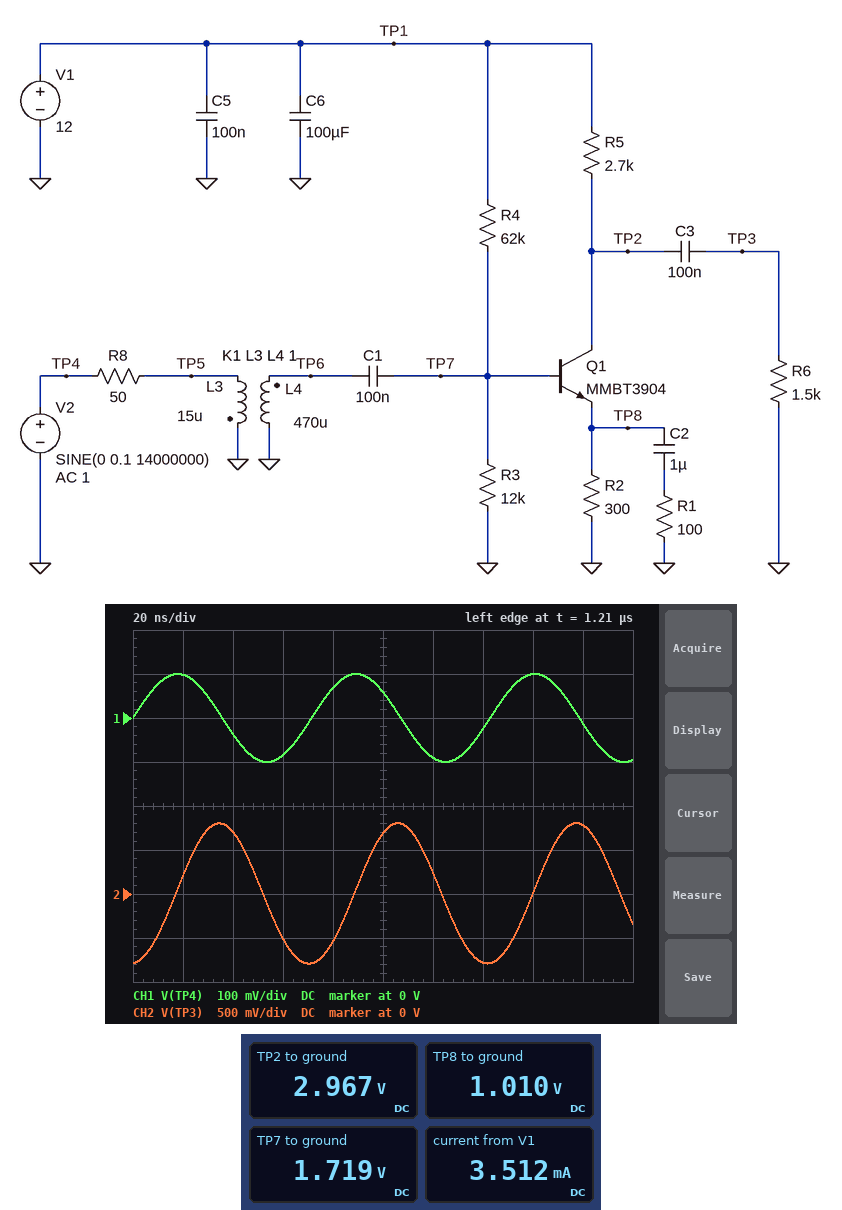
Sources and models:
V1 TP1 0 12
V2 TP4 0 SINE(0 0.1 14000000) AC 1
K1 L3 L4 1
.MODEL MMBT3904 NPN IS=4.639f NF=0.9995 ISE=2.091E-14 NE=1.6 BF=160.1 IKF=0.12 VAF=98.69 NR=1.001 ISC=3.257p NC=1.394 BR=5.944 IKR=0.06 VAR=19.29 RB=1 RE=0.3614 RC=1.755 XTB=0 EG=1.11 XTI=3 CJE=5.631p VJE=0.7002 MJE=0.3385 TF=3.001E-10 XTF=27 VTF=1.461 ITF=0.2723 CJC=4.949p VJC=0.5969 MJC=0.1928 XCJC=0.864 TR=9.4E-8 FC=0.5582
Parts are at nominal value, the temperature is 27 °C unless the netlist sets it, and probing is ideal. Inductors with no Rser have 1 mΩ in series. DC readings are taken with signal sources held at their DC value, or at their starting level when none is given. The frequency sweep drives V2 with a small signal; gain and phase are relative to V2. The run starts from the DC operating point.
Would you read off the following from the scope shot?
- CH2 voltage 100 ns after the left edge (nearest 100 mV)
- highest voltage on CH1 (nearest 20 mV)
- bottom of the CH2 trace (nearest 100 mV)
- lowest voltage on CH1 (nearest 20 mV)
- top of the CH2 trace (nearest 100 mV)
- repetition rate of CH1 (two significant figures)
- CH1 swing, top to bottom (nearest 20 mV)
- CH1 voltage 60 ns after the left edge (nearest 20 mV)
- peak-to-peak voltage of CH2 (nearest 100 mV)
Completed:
700 mV
100 mV
-800 mV
-100 mV
800 mV
14 MHz
200 mV
-80 mV
1.6 V
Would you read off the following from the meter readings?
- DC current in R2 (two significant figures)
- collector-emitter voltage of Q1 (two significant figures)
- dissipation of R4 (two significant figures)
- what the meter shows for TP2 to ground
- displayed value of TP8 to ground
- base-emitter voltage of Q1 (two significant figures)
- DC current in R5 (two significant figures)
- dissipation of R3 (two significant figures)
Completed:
3.4 mA
2.0 V
1.7 mW
2.967 V
1.010 V
710 mV
3.3 mA
250 µW
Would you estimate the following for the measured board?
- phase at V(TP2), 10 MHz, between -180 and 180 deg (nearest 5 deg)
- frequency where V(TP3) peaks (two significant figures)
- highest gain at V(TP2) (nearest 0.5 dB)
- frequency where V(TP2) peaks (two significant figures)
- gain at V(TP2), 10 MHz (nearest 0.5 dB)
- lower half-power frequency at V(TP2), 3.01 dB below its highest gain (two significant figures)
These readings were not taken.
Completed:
-80 deg
970 kHz
34.0 dB
970 kHz
21.0 dB
350 kHz
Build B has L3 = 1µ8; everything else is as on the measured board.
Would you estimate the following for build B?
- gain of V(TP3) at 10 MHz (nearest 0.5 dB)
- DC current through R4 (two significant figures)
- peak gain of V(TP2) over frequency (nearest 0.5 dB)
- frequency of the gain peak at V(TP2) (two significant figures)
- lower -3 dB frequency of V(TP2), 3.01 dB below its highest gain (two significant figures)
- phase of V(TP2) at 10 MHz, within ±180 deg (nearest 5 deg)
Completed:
12.5 dB
170 µA
34.5 dB
990 kHz
670 kHz
-90 deg
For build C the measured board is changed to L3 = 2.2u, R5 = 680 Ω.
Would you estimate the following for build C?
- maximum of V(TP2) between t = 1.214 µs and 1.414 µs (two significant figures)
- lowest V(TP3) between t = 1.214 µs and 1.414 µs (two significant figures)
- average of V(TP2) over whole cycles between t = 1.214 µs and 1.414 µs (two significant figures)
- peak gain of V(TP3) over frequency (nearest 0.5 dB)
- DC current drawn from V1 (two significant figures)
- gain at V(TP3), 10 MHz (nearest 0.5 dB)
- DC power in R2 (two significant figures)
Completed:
10 V
-360 mV
9.7 V
29.0 dB
3.6 mA
14.0 dB
3.5 mW
